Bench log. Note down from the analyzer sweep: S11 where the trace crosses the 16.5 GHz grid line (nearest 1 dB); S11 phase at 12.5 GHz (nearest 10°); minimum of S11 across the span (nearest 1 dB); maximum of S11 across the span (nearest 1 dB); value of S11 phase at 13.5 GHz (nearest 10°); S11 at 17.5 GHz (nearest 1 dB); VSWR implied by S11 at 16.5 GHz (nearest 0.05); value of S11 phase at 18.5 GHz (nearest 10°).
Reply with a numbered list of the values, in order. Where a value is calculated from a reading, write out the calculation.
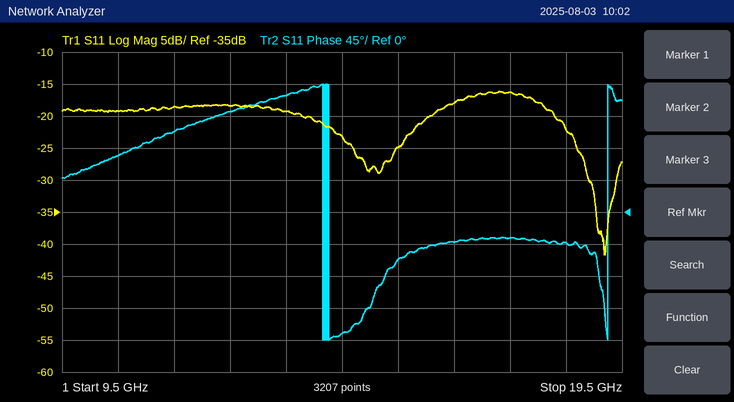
1. -18 dB
2. 140°
3. -42 dB
4. -16 dB
5. 160°
6. -16 dB
7. |Γ| = 10^(-18/20) = 0.1259; VSWR = (1 + 0.1259)/(1 − 0.1259) ≈ 1.29, so 1.30 to the nearest 0.05
8. -40°
